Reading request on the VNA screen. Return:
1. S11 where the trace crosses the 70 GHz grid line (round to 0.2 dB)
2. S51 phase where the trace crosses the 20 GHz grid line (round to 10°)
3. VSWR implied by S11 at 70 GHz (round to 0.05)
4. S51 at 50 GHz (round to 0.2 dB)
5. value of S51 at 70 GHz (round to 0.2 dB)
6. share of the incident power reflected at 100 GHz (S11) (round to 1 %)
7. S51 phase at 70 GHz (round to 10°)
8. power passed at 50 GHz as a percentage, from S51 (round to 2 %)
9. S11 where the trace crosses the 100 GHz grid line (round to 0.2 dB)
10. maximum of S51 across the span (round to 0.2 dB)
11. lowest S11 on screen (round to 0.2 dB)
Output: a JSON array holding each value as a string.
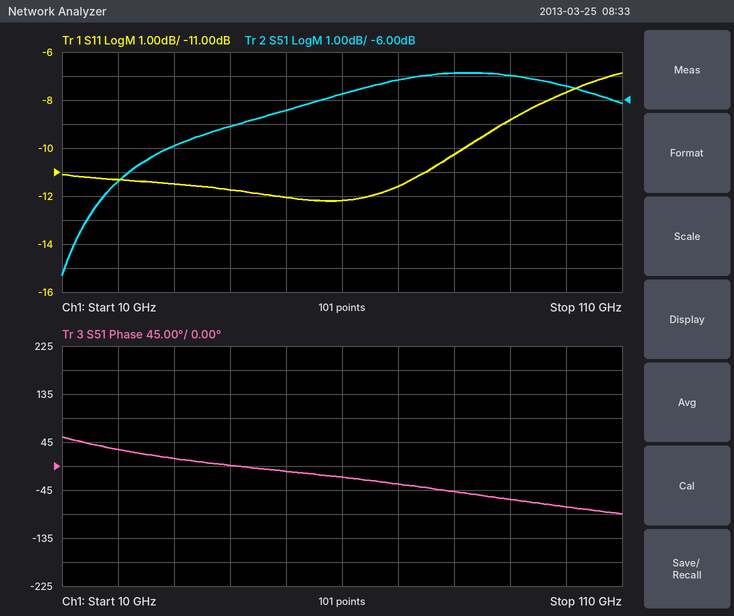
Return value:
["-11.6 dB", "30°", "1.70", "-6.4 dB", "-5.2 dB", "17 %", "-30°", "22 %", "-7.6 dB", "-4.8 dB", "-12.2 dB"]
